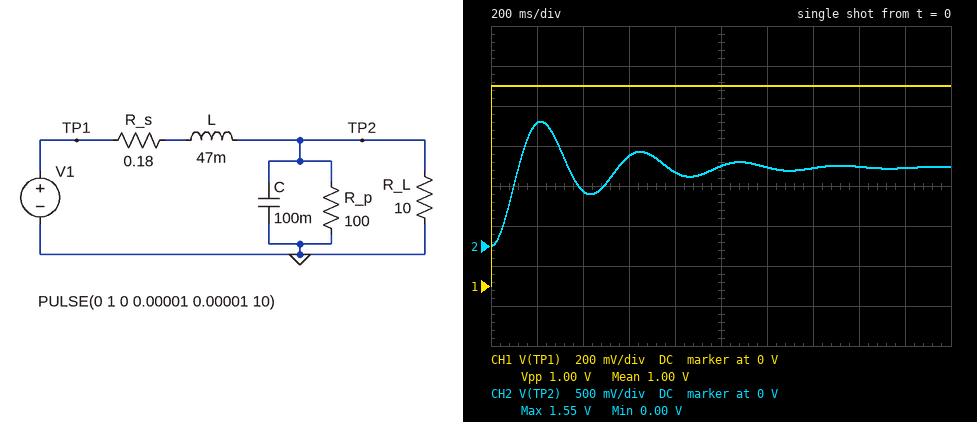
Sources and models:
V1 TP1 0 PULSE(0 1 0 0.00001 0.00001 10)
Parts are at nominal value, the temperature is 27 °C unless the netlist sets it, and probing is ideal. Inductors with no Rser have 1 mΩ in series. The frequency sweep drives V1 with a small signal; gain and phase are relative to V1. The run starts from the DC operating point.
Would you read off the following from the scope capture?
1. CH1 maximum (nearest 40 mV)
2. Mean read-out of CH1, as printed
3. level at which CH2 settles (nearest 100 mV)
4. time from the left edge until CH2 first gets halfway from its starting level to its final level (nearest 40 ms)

1.00 V
1.00 V
1.0 V
80 ms
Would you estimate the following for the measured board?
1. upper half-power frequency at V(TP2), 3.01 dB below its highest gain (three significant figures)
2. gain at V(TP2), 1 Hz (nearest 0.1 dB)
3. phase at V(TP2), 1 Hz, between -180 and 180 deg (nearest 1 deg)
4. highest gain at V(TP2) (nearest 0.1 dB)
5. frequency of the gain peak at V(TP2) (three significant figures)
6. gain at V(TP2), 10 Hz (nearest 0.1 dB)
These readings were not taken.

2.65 Hz
1.4 dB
-10 deg
9.4 dB
2.28 Hz
-24.9 dB
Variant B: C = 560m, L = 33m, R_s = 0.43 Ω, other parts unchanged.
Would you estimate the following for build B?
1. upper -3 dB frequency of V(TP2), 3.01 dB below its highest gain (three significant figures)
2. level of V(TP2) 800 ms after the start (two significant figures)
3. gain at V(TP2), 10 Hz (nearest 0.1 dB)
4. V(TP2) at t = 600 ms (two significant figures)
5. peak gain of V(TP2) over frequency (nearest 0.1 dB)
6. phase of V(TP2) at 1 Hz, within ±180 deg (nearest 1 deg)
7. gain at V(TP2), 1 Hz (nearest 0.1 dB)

921 mHz
960 mV
-37.3 dB
940 mV
-0.4 dB
-78 deg
-3.9 dB
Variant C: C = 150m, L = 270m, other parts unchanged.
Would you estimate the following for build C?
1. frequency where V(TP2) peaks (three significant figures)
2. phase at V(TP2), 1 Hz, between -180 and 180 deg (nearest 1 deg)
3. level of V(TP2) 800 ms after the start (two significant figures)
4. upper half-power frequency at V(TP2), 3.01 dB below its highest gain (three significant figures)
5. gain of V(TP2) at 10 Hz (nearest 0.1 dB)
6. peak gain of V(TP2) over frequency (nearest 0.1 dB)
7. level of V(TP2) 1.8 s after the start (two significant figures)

783 mHz
-148 deg
1.4 V
889 mHz
-44.0 dB
11.0 dB
1.2 V
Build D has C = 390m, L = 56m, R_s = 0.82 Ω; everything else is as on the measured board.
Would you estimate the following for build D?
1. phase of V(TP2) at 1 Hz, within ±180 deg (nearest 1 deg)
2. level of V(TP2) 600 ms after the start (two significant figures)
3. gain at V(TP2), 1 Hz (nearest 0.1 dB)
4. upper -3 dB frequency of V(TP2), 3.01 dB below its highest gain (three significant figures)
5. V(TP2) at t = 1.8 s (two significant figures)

-84 deg
830 mV
-6.3 dB
669 mHz
920 mV
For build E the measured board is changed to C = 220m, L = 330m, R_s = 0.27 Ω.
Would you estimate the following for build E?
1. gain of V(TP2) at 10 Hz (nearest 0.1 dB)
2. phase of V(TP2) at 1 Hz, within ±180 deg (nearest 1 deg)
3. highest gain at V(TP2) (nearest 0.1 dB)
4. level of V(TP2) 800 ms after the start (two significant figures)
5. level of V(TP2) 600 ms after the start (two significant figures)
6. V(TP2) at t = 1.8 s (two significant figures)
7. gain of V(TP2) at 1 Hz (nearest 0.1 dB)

-49.1 dB
-162 deg
9.0 dB
1.5 V
1.3 V
680 mV
-5.7 dB
